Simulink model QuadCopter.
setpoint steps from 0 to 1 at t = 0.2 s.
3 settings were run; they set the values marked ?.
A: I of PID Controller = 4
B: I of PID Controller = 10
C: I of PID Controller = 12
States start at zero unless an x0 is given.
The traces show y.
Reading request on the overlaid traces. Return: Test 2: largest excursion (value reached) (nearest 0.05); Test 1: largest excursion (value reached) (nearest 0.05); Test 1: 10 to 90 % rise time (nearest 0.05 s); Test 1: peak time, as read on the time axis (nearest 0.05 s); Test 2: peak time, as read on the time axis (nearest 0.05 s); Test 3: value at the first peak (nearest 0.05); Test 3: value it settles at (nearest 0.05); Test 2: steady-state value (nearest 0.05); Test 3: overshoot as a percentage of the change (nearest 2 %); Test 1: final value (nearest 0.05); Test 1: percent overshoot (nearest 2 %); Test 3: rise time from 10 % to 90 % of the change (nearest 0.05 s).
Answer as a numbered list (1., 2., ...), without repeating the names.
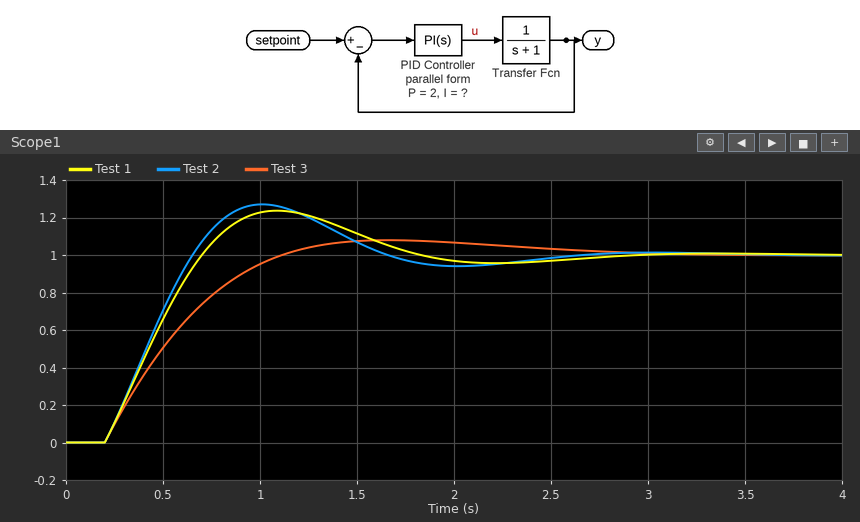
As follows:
1. 1.25
2. 1.25
3. 0.40 s
4. 1.10 s
5. 1.00 s
6. 1.10
7. 1.00
8. 1.00
9. 8 %
10. 1.00
11. 24 %
12. 0.65 s
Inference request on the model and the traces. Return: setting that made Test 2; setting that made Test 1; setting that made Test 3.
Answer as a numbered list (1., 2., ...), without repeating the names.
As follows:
1. C
2. B
3. A
